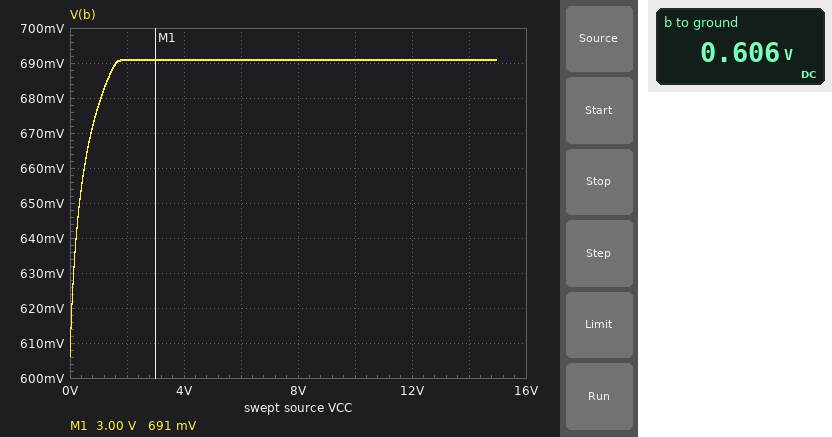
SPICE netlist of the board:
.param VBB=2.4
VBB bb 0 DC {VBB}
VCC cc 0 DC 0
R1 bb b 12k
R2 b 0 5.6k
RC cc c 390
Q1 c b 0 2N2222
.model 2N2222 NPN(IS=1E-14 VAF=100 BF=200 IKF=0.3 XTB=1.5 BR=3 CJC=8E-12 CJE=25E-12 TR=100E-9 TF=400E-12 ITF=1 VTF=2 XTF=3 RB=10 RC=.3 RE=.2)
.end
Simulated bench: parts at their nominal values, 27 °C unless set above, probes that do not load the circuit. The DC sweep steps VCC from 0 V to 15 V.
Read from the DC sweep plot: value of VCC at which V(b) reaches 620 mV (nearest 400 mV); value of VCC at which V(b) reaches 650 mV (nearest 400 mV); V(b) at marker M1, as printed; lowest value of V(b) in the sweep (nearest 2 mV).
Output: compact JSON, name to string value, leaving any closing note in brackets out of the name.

{"value of VCC at which V(b) reaches 620 mV": "0 V", "value of VCC at which V(b) reaches 650 mV": "400 mV", "V(b) at marker M1, as printed": "691 mV", "lowest value of V(b) in the sweep": "606 mV"}
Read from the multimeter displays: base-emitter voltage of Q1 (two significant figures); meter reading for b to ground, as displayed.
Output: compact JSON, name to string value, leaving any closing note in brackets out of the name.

{"base-emitter voltage of Q1": "610 mV", "meter reading for b to ground, as displayed": "0.606 V"}
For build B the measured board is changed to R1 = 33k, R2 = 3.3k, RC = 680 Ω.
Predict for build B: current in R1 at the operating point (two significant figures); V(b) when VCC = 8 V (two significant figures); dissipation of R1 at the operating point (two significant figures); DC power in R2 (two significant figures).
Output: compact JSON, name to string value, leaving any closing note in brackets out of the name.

{"current in R1 at the operating point": "66 µA", "V(b) when VCC = 8 V": "220 mV", "dissipation of R1 at the operating point": "140 µW", "DC power in R2": "14 µW"}
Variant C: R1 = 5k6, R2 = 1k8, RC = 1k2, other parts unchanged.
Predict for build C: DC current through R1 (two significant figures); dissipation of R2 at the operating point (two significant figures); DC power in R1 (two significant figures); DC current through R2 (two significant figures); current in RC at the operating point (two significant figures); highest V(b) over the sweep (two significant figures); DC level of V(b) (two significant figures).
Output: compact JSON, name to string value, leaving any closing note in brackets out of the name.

{"DC current through R1": "330 µA", "dissipation of R2 at the operating point": "180 µW", "DC power in R1": "600 µW", "DC current through R2": "320 µA", "current in RC at the operating point": "4.0 µA", "highest V(b) over the sweep": "580 mV", "DC level of V(b)": "570 mV"}
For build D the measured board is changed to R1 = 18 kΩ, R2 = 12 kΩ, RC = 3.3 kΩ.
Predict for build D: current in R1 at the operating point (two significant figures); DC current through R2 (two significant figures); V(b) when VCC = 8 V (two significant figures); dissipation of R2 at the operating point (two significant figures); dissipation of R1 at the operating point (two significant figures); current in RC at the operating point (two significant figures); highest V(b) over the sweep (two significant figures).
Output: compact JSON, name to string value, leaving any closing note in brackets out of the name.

{"current in R1 at the operating point": "99 µA", "DC current through R2": "51 µA", "V(b) when VCC = 8 V": "680 mV", "dissipation of R2 at the operating point": "31 µW", "dissipation of R1 at the operating point": "180 µW", "current in RC at the operating point": "2.2 µA", "highest V(b) over the sweep": "700 mV"}
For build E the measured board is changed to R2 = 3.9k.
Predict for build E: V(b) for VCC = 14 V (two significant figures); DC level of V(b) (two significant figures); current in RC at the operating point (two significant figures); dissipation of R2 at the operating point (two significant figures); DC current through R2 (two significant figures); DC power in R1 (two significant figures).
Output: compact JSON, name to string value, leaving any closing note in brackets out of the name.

{"V(b) for VCC = 14 V": "590 mV", "DC level of V(b)": "560 mV", "current in RC at the operating point": "6.1 µA", "dissipation of R2 at the operating point": "81 µW", "DC current through R2": "140 µA", "DC power in R1": "280 µW"}
